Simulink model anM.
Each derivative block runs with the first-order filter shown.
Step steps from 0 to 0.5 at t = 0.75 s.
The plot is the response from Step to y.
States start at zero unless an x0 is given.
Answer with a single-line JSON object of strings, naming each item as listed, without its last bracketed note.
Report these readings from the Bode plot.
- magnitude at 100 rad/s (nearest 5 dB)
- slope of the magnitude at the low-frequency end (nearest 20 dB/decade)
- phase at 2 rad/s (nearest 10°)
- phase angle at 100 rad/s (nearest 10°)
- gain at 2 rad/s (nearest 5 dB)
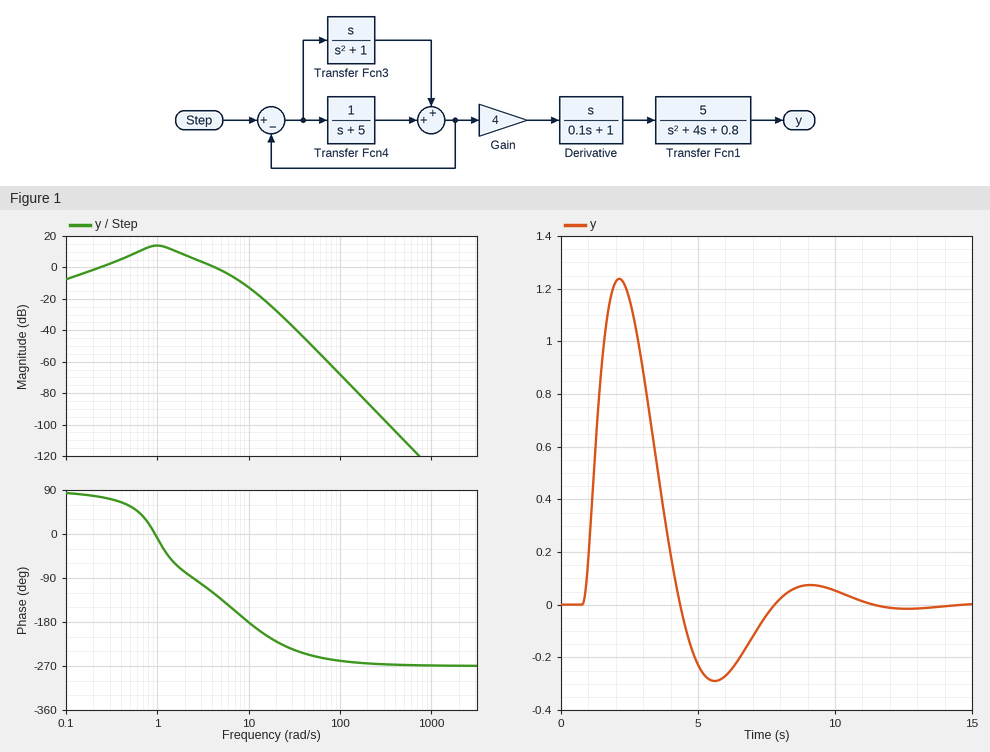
{"magnitude at 100 rad/s": "-70 dB", "slope of the magnitude at the low-frequency end": "20 dB/decade", "phase at 2 rad/s": "-80°", "phase angle at 100 rad/s": "-260°", "gain at 2 rad/s": "10 dB"}
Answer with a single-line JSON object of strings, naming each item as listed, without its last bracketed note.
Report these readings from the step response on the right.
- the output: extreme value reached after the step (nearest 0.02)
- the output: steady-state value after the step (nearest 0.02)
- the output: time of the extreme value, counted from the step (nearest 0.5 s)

{"the output: extreme value reached after the step": "1.24", "the output: steady-state value after the step": "0.00", "the output: time of the extreme value, counted from the step": "1.5 s"}
